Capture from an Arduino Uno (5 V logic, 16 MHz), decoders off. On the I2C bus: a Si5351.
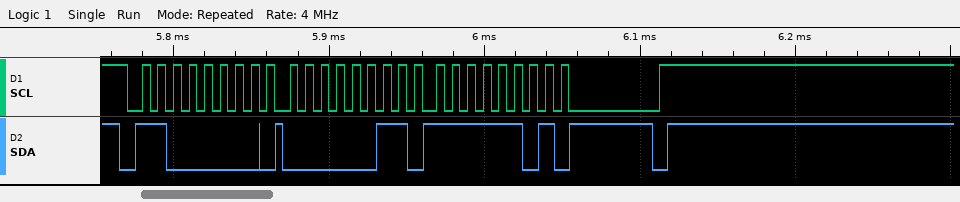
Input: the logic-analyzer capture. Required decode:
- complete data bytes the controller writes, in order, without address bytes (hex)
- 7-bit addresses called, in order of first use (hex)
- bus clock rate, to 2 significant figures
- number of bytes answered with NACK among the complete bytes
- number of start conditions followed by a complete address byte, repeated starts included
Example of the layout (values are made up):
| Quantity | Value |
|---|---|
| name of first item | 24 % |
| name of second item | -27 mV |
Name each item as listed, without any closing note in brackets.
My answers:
| Quantity | Value |
|---|---|
| complete data bytes the controller writes, in order, without address bytes | 03 FD |
| 7-bit addresses called, in order of first use | 0x60 |
| bus clock rate, to 2 significant figures | 100 kHz |
| number of bytes answered with NACK among the complete bytes | 0 |
| number of start conditions followed by a complete address byte, repeated starts included | 1 |
